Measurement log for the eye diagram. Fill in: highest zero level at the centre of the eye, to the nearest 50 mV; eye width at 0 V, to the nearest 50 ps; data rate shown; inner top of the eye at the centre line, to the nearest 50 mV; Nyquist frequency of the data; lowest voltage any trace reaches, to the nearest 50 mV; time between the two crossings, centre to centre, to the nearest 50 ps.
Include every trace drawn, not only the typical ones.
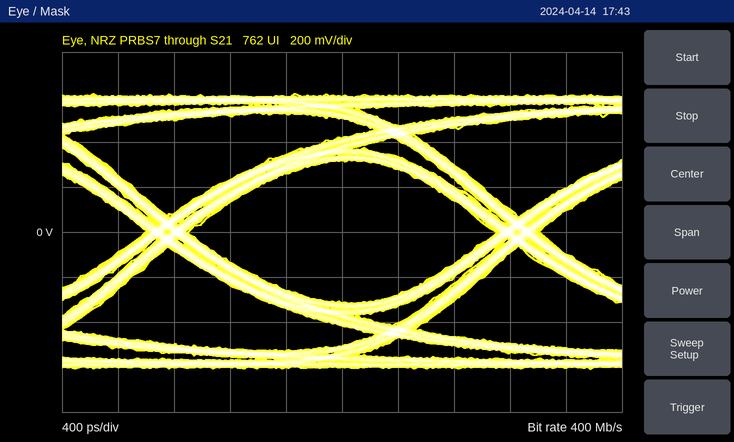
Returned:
-300 mV
2.20 ns
400 Mb/s
300 mV
200 MHz
-600 mV
2.50 ns
